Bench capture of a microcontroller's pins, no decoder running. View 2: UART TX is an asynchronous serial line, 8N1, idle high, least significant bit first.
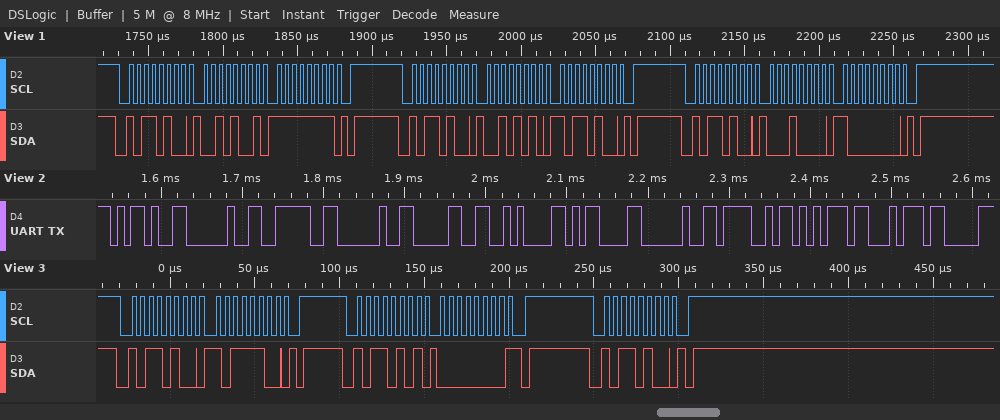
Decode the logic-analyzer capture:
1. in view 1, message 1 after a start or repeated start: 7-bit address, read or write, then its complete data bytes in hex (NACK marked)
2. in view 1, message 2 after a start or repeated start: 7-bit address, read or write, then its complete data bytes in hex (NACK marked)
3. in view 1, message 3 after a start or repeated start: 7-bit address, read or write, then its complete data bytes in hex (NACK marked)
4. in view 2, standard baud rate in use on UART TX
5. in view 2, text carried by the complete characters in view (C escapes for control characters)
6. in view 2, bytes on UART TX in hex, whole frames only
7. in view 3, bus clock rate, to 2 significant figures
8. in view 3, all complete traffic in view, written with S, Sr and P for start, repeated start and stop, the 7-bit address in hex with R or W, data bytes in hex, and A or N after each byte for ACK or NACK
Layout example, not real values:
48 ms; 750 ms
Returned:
0x5A write: 29 FF; 0x5A write: 2A B4; 0x5A write: 10 80; 115200 baud; "- > 0\n\r Out"; 2D 20 3E 20 30 0A 0D 20 4F 75 74; 200 kHz; S 5AW A BC A P S 5AR A 00 N P S 5AW A P
